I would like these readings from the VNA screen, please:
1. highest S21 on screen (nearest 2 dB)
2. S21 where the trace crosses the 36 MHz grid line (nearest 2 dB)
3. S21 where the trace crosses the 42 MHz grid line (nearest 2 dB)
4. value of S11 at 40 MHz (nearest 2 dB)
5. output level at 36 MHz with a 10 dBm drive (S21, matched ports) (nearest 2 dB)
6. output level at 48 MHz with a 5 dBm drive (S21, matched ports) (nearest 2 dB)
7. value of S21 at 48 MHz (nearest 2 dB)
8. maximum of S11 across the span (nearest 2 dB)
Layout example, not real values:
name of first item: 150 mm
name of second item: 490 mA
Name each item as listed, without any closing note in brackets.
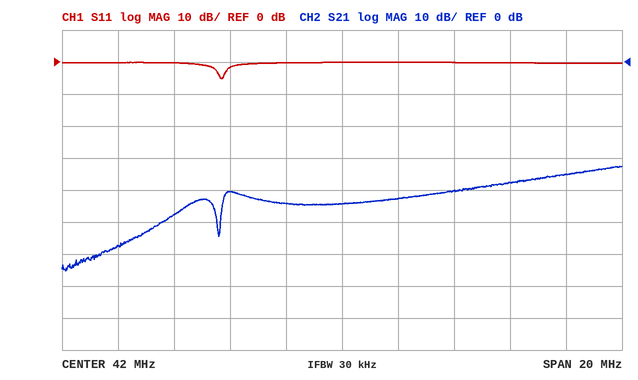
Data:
highest S21 on screen: -32 dB
S21 where the trace crosses the 36 MHz grid line: -48 dB
S21 where the trace crosses the 42 MHz grid line: -44 dB
value of S11 at 40 MHz: 0 dB
output level at 36 MHz with a 10 dBm drive (S21, matched ports): -38 dBm
output level at 48 MHz with a 5 dBm drive (S21, matched ports): -32 dBm
value of S21 at 48 MHz: -38 dB
maximum of S11 across the span: 0 dB
